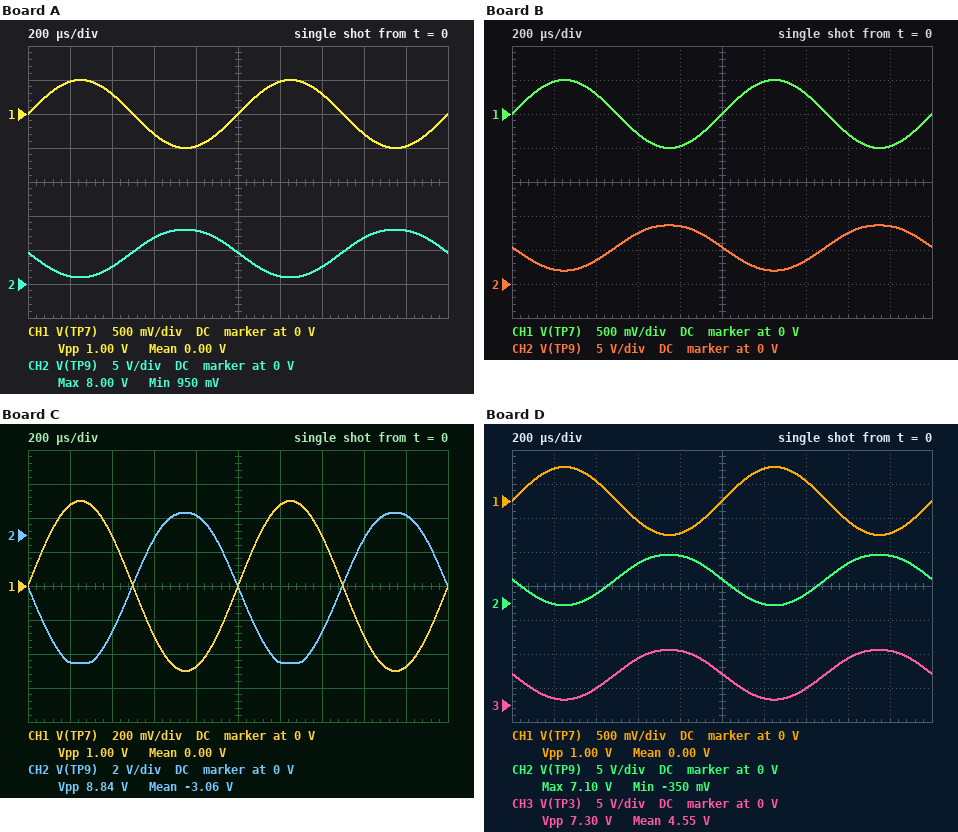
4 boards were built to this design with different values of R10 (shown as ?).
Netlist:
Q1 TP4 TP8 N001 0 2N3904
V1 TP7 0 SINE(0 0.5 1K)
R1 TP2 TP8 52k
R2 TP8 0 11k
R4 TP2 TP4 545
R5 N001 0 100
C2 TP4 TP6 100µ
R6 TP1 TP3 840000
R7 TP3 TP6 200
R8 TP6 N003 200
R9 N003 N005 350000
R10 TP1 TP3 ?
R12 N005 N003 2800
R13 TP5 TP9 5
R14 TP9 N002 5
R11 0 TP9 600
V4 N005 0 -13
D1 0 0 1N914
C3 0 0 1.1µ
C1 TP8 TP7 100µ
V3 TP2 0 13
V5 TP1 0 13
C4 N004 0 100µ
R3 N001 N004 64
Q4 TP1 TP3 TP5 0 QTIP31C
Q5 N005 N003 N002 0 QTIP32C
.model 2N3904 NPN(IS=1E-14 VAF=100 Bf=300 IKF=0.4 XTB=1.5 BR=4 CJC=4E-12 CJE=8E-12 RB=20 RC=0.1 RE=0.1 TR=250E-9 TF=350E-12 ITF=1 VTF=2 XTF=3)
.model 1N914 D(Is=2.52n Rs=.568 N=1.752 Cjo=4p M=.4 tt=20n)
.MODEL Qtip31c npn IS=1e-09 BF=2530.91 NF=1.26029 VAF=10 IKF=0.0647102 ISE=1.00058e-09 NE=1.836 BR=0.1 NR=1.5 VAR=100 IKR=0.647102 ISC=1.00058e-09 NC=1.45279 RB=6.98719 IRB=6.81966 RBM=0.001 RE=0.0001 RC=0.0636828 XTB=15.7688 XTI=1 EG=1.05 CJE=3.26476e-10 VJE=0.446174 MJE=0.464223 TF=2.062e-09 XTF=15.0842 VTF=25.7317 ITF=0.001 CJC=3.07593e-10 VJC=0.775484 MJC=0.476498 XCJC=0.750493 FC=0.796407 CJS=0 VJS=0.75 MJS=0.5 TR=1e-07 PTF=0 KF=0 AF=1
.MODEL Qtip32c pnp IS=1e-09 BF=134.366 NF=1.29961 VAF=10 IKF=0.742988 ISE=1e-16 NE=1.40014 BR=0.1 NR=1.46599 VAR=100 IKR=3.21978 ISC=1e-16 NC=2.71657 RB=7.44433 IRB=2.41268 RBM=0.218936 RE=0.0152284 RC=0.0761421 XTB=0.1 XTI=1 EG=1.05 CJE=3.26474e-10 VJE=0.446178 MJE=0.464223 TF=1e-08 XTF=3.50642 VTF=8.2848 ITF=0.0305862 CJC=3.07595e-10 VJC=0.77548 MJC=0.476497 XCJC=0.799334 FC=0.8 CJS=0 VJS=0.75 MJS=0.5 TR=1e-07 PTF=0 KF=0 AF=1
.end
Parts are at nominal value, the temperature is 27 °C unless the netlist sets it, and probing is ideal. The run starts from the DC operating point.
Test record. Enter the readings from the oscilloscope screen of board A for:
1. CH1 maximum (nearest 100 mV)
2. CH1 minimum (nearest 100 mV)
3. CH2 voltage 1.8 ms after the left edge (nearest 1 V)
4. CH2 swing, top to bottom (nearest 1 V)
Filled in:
500 mV
-500 mV
8 V
7 V
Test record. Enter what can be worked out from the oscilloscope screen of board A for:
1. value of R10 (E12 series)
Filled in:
1.2 kΩ
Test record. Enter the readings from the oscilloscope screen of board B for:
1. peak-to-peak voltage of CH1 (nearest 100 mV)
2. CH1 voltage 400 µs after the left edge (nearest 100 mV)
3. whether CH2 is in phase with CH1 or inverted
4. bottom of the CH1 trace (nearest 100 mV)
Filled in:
1.0 V
300 mV
inverted
-500 mV
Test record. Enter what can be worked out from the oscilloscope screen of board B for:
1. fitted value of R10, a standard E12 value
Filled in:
1 kΩ
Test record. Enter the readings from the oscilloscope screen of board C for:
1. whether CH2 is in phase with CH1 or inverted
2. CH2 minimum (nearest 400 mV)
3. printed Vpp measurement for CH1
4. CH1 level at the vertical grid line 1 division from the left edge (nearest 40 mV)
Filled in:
inverted
-7.6 V
1.00 V
480 mV
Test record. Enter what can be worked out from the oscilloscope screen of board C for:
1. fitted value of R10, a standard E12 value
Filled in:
4.7 kΩ
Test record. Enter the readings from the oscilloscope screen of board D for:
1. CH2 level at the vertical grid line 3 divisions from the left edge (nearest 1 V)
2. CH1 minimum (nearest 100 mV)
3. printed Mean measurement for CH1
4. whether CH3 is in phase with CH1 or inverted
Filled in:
6 V
-500 mV
0.00 V
inverted
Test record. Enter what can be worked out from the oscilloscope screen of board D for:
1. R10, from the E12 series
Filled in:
1.5 kΩ
